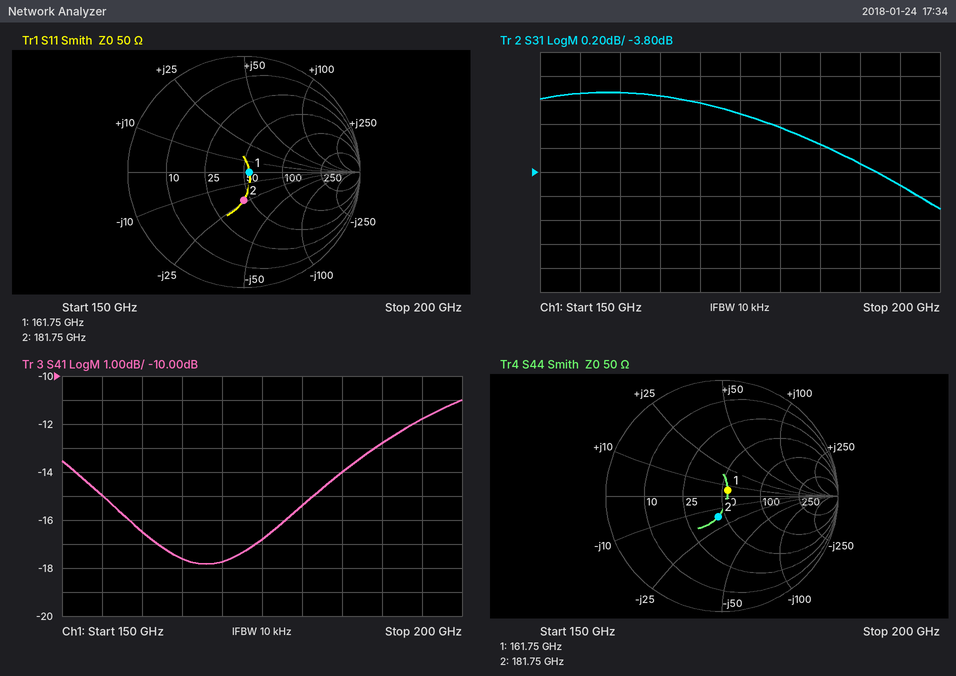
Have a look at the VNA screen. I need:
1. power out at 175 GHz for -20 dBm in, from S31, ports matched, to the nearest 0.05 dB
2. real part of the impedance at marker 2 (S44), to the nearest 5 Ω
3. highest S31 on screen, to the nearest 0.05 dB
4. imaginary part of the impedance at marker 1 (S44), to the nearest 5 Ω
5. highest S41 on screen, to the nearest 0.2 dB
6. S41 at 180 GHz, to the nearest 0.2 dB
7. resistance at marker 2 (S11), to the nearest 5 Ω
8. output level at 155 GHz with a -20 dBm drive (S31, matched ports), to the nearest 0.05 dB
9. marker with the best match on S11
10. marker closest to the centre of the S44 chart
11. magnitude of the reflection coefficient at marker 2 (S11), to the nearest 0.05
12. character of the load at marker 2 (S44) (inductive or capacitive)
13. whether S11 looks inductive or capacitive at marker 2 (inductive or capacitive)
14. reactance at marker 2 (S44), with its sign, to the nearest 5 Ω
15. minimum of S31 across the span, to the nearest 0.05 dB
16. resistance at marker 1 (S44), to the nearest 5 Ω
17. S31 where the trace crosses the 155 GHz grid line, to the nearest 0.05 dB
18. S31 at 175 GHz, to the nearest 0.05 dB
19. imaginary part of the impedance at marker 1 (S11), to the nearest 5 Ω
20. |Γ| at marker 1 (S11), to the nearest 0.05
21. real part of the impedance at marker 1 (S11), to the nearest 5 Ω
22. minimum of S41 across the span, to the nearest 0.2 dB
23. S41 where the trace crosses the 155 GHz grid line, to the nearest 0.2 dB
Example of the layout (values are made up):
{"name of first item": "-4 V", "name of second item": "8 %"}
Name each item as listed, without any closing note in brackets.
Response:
{"power out at 175 GHz for -20 dBm in, from S31, ports matched, to the nearest 0.05 dB": "-23.30 dBm", "real part of the impedance at marker 2 (S44), to the nearest 5 Ω": "45 Ω", "highest S31 on screen, to the nearest 0.05 dB": "-3.15 dB", "imaginary part of the impedance at marker 1 (S44), to the nearest 5 Ω": "+5 Ω", "highest S41 on screen, to the nearest 0.2 dB": "-11.0 dB", "S41 at 180 GHz, to the nearest 0.2 dB": "-15.4 dB", "resistance at marker 2 (S11), to the nearest 5 Ω": "45 Ω", "output level at 155 GHz with a -20 dBm drive (S31, matched ports), to the nearest 0.05 dB": "-23.15 dBm", "marker with the best match on S11": "marker 1", "marker closest to the centre of the S44 chart": "marker 1", "magnitude of the reflection coefficient at marker 2 (S11), to the nearest 0.05": "0.25", "character of the load at marker 2 (S44)": "capacitive", "whether S11 looks inductive or capacitive at marker 2": "capacitive", "reactance at marker 2 (S44), with its sign, to the nearest 5 Ω": "-15 Ω", "minimum of S31 across the span, to the nearest 0.05 dB": "-4.10 dB", "resistance at marker 1 (S44), to the nearest 5 Ω": "55 Ω", "S31 where the trace crosses the 155 GHz grid line, to the nearest 0.05 dB": "-3.15 dB", "S31 at 175 GHz, to the nearest 0.05 dB": "-3.30 dB", "imaginary part of the impedance at marker 1 (S11), to the nearest 5 Ω": "0 Ω", "|Γ| at marker 1 (S11), to the nearest 0.05": "0.05", "real part of the impedance at marker 1 (S11), to the nearest 5 Ω": "55 Ω", "minimum of S41 across the span, to the nearest 0.2 dB": "-17.8 dB", "S41 where the trace crosses the 155 GHz grid line, to the nearest 0.2 dB": "-15.0 dB"}
